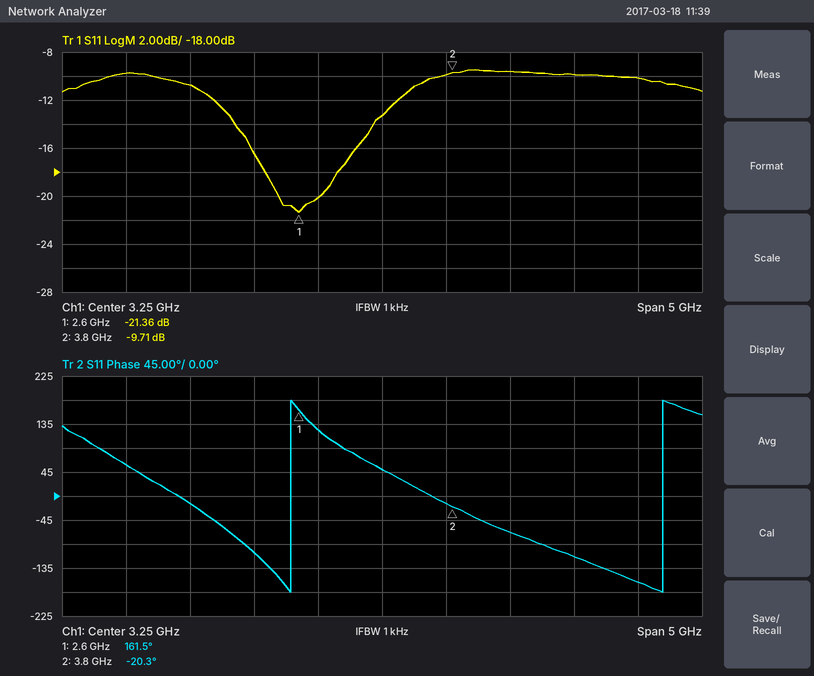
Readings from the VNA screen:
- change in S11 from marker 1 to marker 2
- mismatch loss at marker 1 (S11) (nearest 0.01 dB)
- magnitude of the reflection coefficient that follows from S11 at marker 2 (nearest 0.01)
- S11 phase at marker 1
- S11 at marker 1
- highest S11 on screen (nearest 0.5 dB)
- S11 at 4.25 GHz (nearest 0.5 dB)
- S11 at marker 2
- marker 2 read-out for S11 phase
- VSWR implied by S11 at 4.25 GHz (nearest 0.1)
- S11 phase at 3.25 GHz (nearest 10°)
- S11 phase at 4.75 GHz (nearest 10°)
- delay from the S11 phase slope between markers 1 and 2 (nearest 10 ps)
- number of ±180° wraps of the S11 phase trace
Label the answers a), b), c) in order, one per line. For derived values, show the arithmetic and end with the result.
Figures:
a) -9.71 − (-21.36) = 11.65 dB
b) −10 log10(1 − 10^(-21.36/10)) ≈ 0.03 dB
c) 10^(-9.71/20) ≈ 0.33
d) 161.5°
e) -21.36 dB
f) -9.5 dB
g) -9.5 dB
h) -9.71 dB
i) -20.3°
j) |Γ| = 10^(-9.5/20) = 0.3350; VSWR = (1 + 0.3350)/(1 − 0.3350) ≈ 2.0
k) 50°
l) -110°
m) −(-20.3° − (161.5°))/(360° × 1.2 GHz) ≈ 421 ps, so 420 ps to the nearest 10 ps
n) 2
